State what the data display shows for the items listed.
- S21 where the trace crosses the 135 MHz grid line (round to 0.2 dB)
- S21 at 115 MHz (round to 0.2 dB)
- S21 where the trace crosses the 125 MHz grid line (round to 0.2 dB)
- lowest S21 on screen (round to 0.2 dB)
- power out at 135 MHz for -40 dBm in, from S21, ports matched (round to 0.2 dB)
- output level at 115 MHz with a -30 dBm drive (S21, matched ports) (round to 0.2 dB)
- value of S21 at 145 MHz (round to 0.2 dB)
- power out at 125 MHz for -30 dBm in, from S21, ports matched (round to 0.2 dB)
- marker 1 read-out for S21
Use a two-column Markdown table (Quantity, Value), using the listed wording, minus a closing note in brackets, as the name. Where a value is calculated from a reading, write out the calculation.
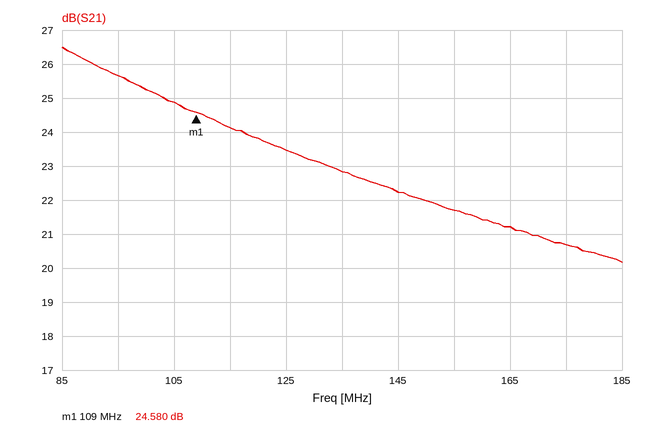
| Quantity | Value |
|---|---|
| S21 where the trace crosses the 135 MHz grid line | 22.8 dB |
| S21 at 115 MHz | 24.2 dB |
| S21 where the trace crosses the 125 MHz grid line | 23.4 dB |
| lowest S21 on screen | 20.2 dB |
| power out at 135 MHz for -40 dBm in, from S21, ports matched | -40 dBm + (22.8 dB) = -17.2 dBm |
| output level at 115 MHz with a -30 dBm drive (S21, matched ports) | -30 dBm + (24.2 dB) = -5.8 dBm |
| value of S21 at 145 MHz | 22.2 dB |
| power out at 125 MHz for -30 dBm in, from S21, ports matched | -30 dBm + (23.4 dB) = -6.6 dBm |
| marker 1 read-out for S21 | 24.580 dB |
